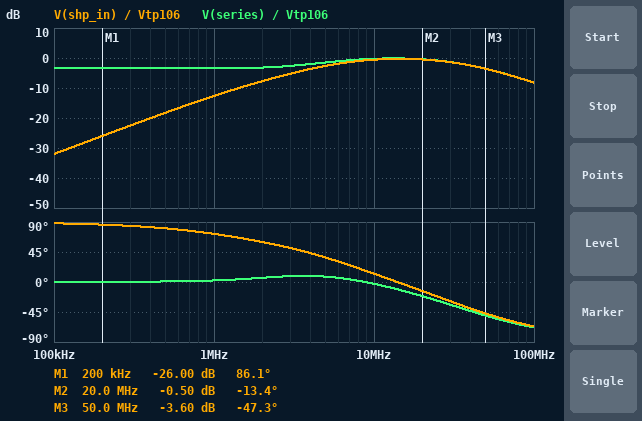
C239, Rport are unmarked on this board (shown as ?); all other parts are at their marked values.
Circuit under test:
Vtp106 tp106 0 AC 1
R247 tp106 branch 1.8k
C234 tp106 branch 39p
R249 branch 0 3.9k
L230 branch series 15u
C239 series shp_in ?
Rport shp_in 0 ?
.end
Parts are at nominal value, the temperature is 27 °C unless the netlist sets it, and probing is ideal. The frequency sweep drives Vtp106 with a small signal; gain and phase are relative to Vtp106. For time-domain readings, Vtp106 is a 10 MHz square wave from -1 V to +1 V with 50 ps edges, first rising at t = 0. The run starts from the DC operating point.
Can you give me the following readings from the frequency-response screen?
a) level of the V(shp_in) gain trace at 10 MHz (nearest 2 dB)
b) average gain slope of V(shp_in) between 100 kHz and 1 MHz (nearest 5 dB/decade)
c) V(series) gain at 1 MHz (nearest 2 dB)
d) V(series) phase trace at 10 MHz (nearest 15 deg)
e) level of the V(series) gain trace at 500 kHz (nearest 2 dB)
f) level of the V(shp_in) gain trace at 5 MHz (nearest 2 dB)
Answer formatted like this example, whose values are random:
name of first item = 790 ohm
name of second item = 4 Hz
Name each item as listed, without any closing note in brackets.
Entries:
level of the V(shp_in) gain trace at 10 MHz = 0 dB
average gain slope of V(shp_in) between 100 kHz and 1 MHz = 20 dB/decade
V(series) gain at 1 MHz = -4 dB
V(series) phase trace at 10 MHz = 0 deg
level of the V(series) gain trace at 500 kHz = -4 dB
level of the V(shp_in) gain trace at 5 MHz = -2 dB
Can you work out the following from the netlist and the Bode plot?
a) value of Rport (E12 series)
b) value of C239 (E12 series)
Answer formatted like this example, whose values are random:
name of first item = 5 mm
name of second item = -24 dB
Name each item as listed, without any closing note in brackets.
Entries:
value of Rport = 3.9 kΩ
value of C239 = 15 pF
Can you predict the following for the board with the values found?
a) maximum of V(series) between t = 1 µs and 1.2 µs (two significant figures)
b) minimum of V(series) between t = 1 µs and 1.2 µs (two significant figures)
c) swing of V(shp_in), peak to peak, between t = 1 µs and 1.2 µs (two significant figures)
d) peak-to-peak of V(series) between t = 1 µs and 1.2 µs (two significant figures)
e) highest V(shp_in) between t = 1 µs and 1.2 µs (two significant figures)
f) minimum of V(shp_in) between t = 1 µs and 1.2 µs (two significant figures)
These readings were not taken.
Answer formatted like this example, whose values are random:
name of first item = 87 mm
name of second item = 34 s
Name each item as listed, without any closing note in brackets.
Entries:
maximum of V(series) between t = 1 µs and 1.2 µs = 1.1 V
minimum of V(series) between t = 1 µs and 1.2 µs = -1.1 V
swing of V(shp_in), peak to peak, between t = 1 µs and 1.2 µs = 2.6 V
peak-to-peak of V(series) between t = 1 µs and 1.2 µs = 2.3 V
highest V(shp_in) between t = 1 µs and 1.2 µs = 1.3 V
minimum of V(shp_in) between t = 1 µs and 1.2 µs = -1.3 V
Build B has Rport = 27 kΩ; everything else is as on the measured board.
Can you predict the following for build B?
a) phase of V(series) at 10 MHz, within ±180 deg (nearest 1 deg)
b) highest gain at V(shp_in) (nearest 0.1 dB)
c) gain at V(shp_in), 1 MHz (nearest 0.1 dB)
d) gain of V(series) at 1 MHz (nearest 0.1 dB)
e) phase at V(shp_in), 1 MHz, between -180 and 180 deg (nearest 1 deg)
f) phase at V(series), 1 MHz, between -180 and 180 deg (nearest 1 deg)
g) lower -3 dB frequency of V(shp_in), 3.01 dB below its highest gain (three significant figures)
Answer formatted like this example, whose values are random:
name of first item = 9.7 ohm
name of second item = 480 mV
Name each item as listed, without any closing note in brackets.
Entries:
phase of V(series) at 10 MHz, within ±180 deg = 4 deg
highest gain at V(shp_in) = -0.1 dB
gain at V(shp_in), 1 MHz = -3.9 dB
gain of V(series) at 1 MHz = -3.2 dB
phase at V(shp_in), 1 MHz, between -180 and 180 deg = 28 deg
phase at V(series), 1 MHz, between -180 and 180 deg = 7 deg
lower -3 dB frequency of V(shp_in), 3.01 dB below its highest gain = 1.56 MHz
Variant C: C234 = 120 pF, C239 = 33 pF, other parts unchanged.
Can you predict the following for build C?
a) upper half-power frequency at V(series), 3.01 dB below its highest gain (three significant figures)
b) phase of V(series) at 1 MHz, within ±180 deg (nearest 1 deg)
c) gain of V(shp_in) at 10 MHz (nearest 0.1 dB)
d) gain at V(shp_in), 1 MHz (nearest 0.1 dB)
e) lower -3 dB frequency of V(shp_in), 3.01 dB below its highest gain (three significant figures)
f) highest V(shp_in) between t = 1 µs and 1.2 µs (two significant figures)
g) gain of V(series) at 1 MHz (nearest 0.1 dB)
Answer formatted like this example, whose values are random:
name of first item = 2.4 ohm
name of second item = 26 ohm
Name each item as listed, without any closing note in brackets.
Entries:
upper half-power frequency at V(series), 3.01 dB below its highest gain = 42.8 MHz
phase of V(series) at 1 MHz, within ±180 deg = 9 deg
gain of V(shp_in) at 10 MHz = -0.1 dB
gain at V(shp_in), 1 MHz = -6.6 dB
lower -3 dB frequency of V(shp_in), 3.01 dB below its highest gain = 1.83 MHz
highest V(shp_in) between t = 1 µs and 1.2 µs = 1.1 V
gain of V(series) at 1 MHz = -2.5 dB
